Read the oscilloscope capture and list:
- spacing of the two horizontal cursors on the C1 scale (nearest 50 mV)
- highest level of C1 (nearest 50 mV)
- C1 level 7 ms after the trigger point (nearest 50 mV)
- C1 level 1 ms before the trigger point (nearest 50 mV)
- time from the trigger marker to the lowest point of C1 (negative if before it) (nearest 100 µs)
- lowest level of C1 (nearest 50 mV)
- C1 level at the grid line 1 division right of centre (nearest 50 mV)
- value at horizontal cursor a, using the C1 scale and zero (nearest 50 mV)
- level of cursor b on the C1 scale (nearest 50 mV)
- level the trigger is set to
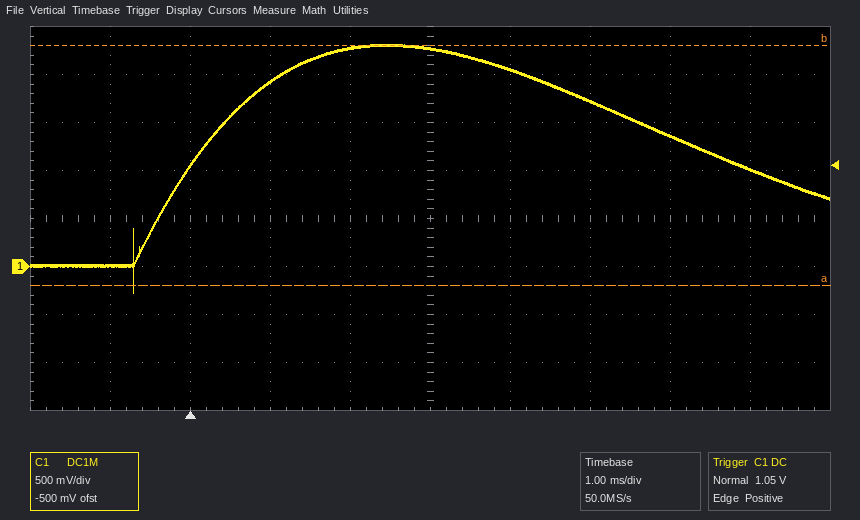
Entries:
2.50 V
2.30 V
1.00 V
0 mV
-700 µs
-250 mV
2.05 V
-200 mV
2.30 V
1.05 V
